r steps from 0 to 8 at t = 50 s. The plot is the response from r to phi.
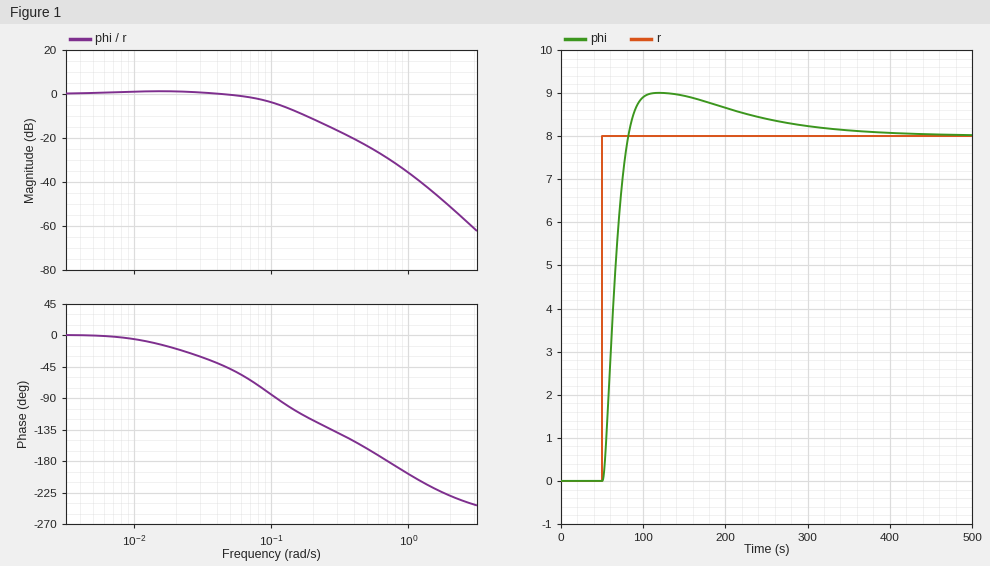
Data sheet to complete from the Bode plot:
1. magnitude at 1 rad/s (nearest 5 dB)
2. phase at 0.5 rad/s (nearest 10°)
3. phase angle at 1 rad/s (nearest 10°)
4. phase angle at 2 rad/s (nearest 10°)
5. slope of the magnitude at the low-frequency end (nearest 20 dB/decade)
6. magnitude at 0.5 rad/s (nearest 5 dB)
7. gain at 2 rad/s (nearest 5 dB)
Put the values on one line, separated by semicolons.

-35 dB; -160°; -200°; -230°; 0 dB/decade; -25 dB; -50 dB
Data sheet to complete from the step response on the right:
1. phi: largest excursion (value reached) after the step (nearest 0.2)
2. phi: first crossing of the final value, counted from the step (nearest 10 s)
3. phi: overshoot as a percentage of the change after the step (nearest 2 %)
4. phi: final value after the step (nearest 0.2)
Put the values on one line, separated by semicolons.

9.0; 30 s; 12 %; 8.0
